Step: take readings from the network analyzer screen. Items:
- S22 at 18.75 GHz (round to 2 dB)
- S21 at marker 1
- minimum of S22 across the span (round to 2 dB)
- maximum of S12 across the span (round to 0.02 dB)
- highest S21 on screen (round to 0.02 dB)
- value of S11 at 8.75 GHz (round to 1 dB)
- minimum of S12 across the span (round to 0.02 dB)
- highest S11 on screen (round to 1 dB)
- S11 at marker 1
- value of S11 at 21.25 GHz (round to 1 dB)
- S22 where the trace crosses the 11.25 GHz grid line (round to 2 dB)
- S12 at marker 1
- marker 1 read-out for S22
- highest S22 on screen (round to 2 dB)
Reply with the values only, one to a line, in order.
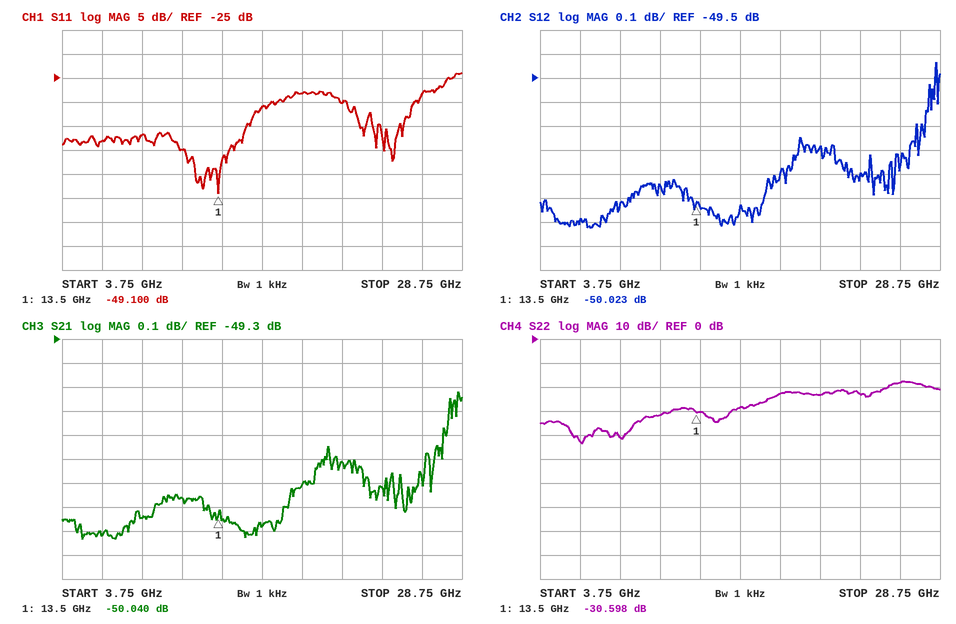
-22 dB
-50.040 dB
-44 dB
-49.44 dB
-49.52 dB
-37 dB
-50.12 dB
-24 dB
-49.100 dB
-30 dB
-32 dB
-50.023 dB
-30.598 dB
-18 dB
